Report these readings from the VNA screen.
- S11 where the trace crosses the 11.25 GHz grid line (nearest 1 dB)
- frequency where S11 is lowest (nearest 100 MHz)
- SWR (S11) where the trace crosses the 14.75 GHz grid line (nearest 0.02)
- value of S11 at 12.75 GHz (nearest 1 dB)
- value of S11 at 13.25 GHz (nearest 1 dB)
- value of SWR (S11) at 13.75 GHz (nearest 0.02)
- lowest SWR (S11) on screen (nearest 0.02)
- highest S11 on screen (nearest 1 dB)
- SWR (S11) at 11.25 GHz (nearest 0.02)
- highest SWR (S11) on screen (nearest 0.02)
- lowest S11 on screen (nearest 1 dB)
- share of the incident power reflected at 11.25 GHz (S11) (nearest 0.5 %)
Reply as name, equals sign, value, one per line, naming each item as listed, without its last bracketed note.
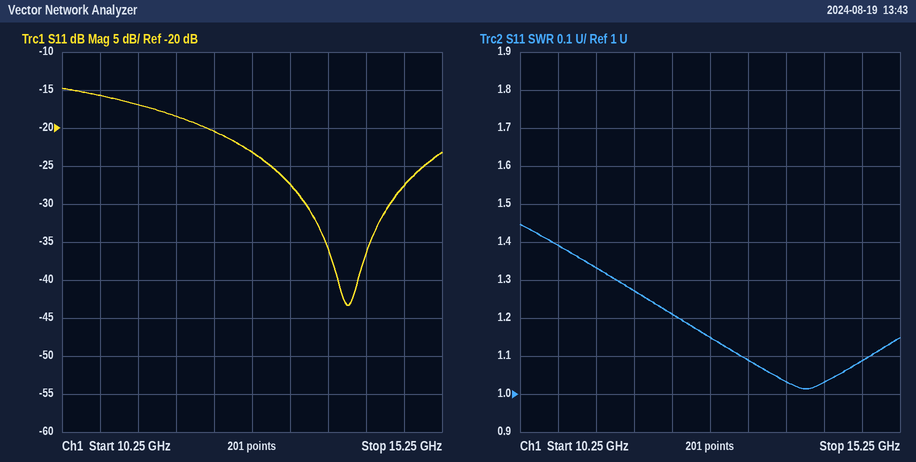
S11 where the trace crosses the 11.25 GHz grid line = -17 dB
frequency where S11 is lowest = 14.0 GHz
SWR (S11) where the trace crosses the 14.75 GHz grid line = 1.08
value of S11 at 12.75 GHz = -23 dB
value of S11 at 13.25 GHz = -27 dB
value of SWR (S11) at 13.75 GHz = 1.04
lowest SWR (S11) on screen = 1.02
highest S11 on screen = -15 dB
SWR (S11) at 11.25 GHz = 1.34
highest SWR (S11) on screen = 1.44
lowest S11 on screen = -43 dB
share of the incident power reflected at 11.25 GHz (S11) = 2.0 %
